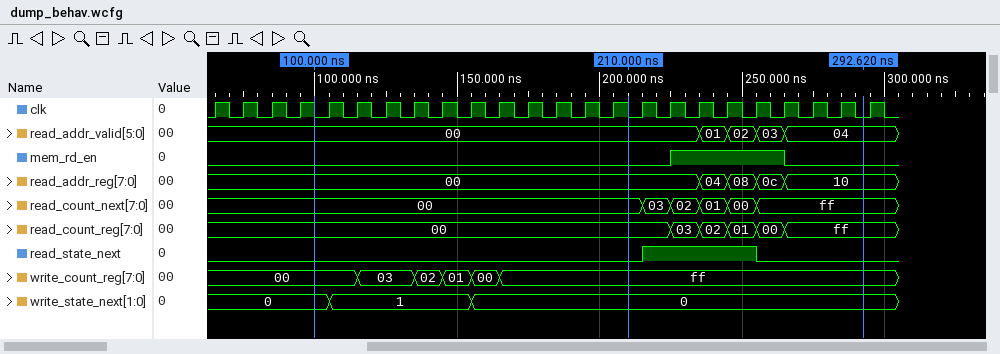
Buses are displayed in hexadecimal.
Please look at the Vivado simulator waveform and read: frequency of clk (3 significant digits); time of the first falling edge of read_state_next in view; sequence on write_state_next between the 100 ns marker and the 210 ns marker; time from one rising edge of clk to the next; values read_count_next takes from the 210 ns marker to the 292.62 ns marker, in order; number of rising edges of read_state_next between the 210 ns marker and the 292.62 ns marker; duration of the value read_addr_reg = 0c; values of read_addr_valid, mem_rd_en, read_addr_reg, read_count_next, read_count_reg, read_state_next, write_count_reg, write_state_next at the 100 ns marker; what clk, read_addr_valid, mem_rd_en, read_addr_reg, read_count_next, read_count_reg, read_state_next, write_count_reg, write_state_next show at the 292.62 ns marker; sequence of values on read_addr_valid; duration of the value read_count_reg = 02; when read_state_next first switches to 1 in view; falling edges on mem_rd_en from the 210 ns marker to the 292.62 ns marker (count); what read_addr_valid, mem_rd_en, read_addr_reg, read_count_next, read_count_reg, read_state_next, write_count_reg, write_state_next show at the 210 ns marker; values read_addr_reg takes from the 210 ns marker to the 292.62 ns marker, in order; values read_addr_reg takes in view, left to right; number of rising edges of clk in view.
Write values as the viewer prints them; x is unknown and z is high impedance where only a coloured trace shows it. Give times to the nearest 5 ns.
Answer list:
100 MHz
255 ns
0, 1, 0
10 ns
00, 03, 02, 01, 00, ff
1
10 ns
read_addr_valid=00, mem_rd_en=0, read_addr_reg=00, read_count_next=00, read_count_reg=00, read_state_next=0, write_count_reg=00, write_state_next=0
clk=0, read_addr_valid=04, mem_rd_en=0, read_addr_reg=10, read_count_next=ff, read_count_reg=ff, read_state_next=0, write_count_reg=ff, write_state_next=0
00, 01, 02, 03, 04
10 ns
215 ns
1
read_addr_valid=00, mem_rd_en=0, read_addr_reg=00, read_count_next=00, read_count_reg=00, read_state_next=0, write_count_reg=ff, write_state_next=0
00, 04, 08, 0c, 10
00, 04, 08, 0c, 10
24
